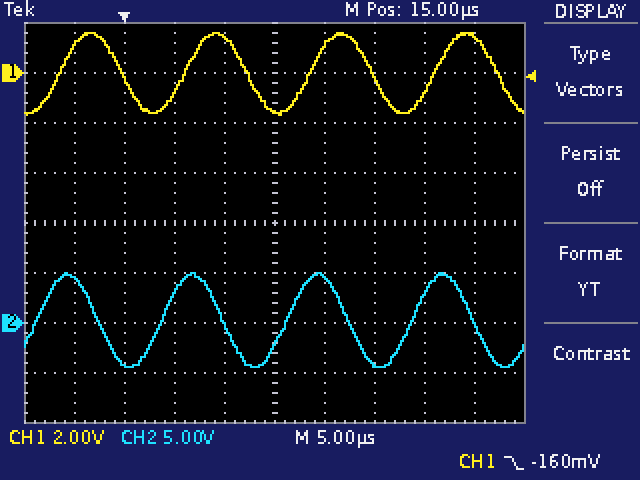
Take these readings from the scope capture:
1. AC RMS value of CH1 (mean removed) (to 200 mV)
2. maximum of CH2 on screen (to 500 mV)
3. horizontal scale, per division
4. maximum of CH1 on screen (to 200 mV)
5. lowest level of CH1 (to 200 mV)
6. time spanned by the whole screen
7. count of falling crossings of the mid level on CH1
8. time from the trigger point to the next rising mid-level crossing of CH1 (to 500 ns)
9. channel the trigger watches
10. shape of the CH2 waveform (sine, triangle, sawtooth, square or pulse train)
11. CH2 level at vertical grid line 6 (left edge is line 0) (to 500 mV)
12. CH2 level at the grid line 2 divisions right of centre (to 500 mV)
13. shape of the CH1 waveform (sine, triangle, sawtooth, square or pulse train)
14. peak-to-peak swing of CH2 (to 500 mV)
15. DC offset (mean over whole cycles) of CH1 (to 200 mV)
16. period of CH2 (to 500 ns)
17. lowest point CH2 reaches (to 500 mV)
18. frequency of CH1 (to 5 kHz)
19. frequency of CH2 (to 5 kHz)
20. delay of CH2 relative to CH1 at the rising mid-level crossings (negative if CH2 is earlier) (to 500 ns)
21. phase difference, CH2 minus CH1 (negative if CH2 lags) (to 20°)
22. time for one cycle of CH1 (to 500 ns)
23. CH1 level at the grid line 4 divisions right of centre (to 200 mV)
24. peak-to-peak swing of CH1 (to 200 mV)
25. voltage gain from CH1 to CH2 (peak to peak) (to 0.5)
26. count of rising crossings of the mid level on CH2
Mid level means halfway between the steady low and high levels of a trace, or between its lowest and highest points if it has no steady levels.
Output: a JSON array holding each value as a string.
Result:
["1.2 V", "5.0 V", "5 µs", "1.6 V", "-1.6 V", "50 µs", "4", "6.0 µs", "CH1", "sine", "4.5 V", "-4.0 V", "sine", "9.5 V", "0.0 V", "12.5 µs", "-4.5 V", "80 kHz", "80 kHz", "-2.0 µs", "+60°", "12.5 µs", "1.4 V", "3.2 V", "3.0", "4"]
